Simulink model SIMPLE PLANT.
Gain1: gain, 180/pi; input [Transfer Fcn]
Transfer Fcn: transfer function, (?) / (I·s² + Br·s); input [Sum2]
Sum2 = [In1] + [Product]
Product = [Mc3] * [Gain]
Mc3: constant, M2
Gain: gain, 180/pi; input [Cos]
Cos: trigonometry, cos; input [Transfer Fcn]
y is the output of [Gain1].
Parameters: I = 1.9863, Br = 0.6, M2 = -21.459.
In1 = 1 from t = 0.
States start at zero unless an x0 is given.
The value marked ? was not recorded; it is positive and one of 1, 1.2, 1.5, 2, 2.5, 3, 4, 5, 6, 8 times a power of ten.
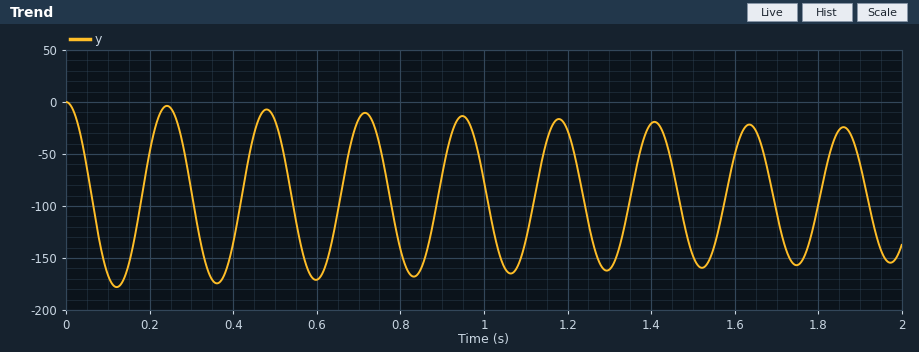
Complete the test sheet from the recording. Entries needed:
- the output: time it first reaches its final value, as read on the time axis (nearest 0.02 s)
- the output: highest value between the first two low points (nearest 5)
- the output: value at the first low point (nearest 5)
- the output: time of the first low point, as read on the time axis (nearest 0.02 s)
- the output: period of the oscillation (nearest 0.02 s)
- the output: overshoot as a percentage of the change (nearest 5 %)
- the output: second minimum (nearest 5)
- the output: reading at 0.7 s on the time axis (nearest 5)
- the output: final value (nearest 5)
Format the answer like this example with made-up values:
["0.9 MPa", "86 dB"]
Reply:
["0.06 s", "-5", "-180", "0.12 s", "0.24 s", "85 %", "-175", "-15", "-95"]
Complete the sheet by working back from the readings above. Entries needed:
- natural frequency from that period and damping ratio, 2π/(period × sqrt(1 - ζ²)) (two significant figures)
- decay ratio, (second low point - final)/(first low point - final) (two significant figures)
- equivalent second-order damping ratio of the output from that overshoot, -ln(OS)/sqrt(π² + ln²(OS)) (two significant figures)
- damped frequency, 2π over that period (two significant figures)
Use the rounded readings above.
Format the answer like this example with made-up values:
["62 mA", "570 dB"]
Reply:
["26 rad/s", "0.94", "0.052", "26 rad/s"]
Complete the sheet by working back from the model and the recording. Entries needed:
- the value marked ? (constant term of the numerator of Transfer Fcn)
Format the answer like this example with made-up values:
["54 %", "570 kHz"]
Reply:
["1.5"]
